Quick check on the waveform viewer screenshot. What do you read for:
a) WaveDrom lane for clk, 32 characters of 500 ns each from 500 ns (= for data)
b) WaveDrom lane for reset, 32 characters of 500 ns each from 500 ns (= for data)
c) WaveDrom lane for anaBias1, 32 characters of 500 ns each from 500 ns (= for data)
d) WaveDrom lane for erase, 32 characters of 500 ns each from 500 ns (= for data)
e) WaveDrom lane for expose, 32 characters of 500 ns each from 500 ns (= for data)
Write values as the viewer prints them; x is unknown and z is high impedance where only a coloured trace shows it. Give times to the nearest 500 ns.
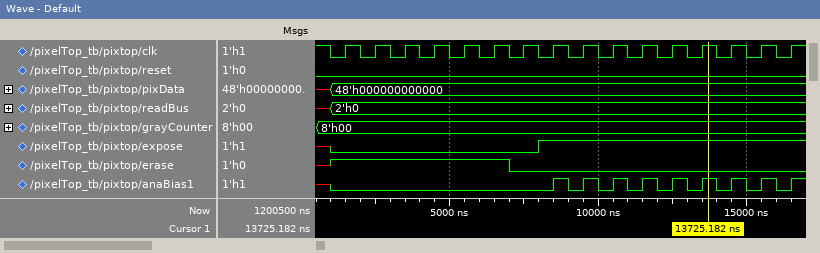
{name: 'clk', wave: '10101010101010101010101010101010'}
{name: 'reset', wave: '0...............................'}
{name: 'anaBias1', wave: 'x0..............1010101010101010'}
{name: 'erase', wave: 'x1...........0..................'}
{name: 'expose', wave: 'x0.............1................'}
